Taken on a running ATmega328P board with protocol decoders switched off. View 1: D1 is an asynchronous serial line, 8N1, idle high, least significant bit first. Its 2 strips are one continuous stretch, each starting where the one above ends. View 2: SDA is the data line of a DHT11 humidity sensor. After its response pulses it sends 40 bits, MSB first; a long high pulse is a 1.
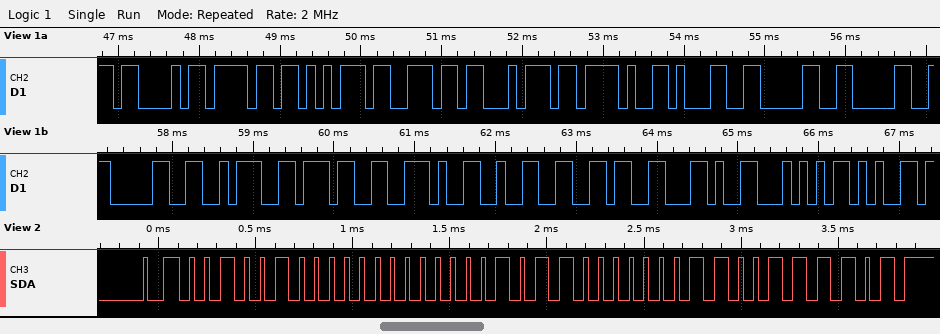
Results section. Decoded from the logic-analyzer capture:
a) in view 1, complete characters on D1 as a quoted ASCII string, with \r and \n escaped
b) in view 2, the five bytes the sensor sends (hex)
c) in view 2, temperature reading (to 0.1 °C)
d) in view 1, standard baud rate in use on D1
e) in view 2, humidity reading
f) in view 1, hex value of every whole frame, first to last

"Count/1000:7.26,Te"
24 00 16 03 3D
22.3 °C
9600 baud
36 %
43 6F 75 6E 74 2F 31 30 30 30 3A 37 2E 32 36 2C 54 65
